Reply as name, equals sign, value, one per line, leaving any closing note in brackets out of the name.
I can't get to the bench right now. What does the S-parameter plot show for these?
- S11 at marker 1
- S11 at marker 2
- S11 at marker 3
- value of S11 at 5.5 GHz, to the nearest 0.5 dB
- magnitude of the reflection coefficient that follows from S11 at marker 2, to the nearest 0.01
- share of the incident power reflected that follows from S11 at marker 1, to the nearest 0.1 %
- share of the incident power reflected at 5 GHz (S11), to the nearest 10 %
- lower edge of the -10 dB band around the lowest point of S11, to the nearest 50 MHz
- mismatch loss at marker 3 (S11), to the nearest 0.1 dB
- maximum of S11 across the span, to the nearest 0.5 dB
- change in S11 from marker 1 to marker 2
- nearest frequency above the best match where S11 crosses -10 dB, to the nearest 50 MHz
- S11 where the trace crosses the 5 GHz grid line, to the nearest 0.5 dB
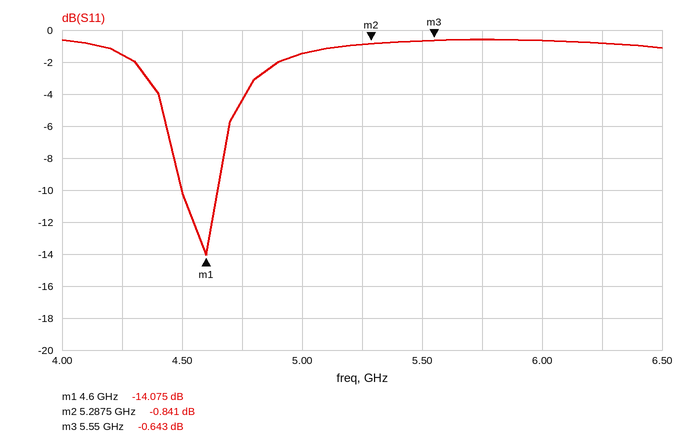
S11 at marker 1 = -14.075 dB
S11 at marker 2 = -0.841 dB
S11 at marker 3 = -0.643 dB
value of S11 at 5.5 GHz, to the nearest 0.5 dB = -0.5 dB
magnitude of the reflection coefficient that follows from S11 at marker 2, to the nearest 0.01 = 0.91
share of the incident power reflected that follows from S11 at marker 1, to the nearest 0.1 % = 3.9 %
share of the incident power reflected at 5 GHz (S11), to the nearest 10 % = 70 %
lower edge of the -10 dB band around the lowest point of S11, to the nearest 50 MHz = 4.50 GHz
mismatch loss at marker 3 (S11), to the nearest 0.1 dB = 8.6 dB
maximum of S11 across the span, to the nearest 0.5 dB = -0.5 dB
change in S11 from marker 1 to marker 2 = 13.234 dB
nearest frequency above the best match where S11 crosses -10 dB, to the nearest 50 MHz = 4.65 GHz
S11 where the trace crosses the 5 GHz grid line, to the nearest 0.5 dB = -1.5 dB
